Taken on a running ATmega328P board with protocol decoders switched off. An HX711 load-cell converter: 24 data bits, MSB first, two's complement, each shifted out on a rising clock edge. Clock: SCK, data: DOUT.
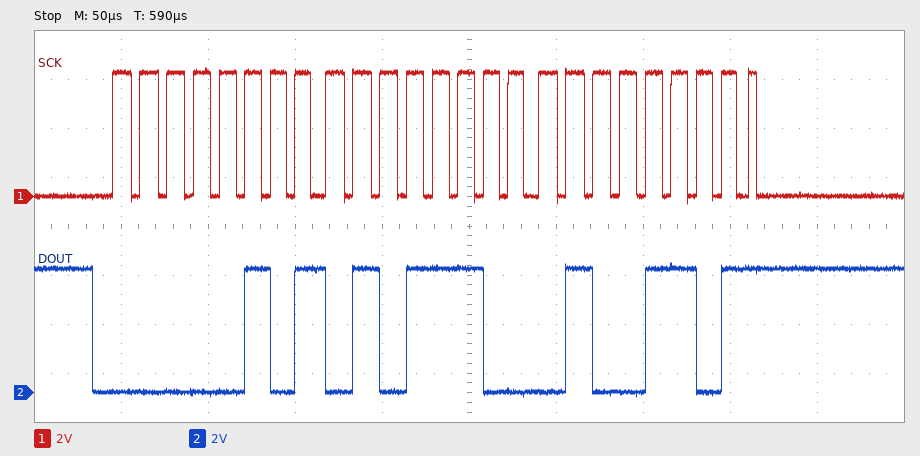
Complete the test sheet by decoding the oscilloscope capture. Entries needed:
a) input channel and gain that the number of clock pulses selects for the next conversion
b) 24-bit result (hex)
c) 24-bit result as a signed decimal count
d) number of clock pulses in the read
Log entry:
channel A, gain 128
0x055C4D
351309
25
